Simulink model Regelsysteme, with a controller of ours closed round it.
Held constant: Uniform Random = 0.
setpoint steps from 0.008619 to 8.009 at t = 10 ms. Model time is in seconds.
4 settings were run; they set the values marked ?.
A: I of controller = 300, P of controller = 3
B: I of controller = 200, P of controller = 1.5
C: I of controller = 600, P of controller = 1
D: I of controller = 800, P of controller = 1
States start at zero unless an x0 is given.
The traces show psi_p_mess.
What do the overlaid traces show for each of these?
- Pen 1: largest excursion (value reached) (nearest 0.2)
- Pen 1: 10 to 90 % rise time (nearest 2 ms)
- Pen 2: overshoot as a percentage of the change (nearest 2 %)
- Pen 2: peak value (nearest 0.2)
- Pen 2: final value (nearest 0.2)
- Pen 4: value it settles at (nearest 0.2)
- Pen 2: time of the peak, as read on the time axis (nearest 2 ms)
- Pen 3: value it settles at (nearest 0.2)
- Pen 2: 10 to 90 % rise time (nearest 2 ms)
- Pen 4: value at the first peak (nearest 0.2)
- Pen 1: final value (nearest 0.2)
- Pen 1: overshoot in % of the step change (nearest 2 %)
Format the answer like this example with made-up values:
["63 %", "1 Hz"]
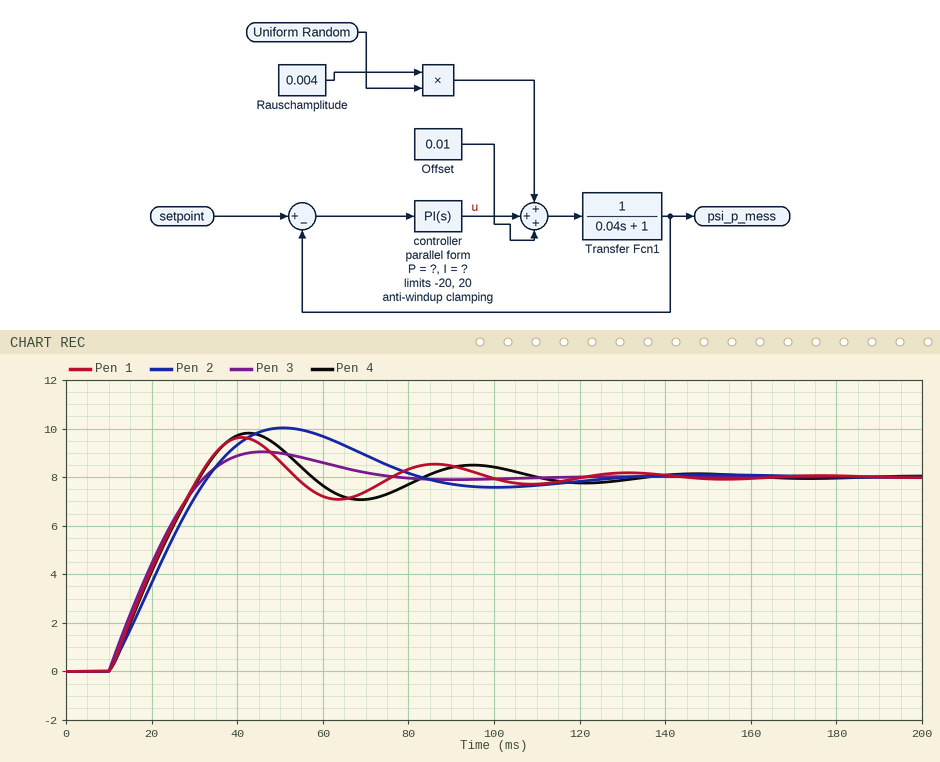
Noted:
["9.6", "16 ms", "26 %", "10.0", "8.0", "8.0", "50 ms", "8.0", "18 ms", "9.8", "8.0", "20 %"]
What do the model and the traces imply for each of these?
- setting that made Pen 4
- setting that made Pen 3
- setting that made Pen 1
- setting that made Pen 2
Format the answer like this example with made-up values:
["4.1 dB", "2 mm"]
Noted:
["C", "A", "D", "B"]
